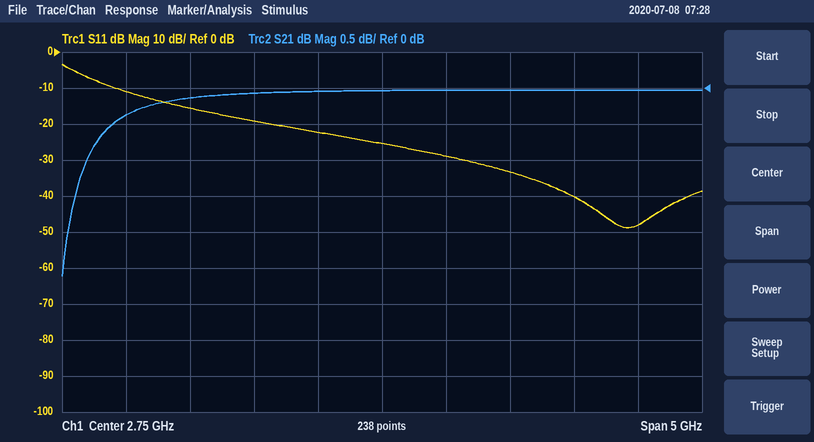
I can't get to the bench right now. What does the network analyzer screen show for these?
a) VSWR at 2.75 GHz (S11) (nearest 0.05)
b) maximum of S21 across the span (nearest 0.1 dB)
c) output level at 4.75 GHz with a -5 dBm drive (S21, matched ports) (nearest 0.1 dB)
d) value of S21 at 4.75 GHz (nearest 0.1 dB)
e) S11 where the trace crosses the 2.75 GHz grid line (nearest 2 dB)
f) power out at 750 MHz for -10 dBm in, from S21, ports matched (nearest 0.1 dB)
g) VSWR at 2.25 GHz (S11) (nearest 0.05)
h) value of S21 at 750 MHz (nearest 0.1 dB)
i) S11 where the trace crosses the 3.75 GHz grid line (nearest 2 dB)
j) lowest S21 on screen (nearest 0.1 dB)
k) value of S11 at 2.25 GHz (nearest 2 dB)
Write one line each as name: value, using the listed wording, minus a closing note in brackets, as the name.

VSWR at 2.75 GHz (S11): 1.10
maximum of S21 across the span: 0.0 dB
output level at 4.75 GHz with a -5 dBm drive (S21, matched ports): -5.0 dBm
value of S21 at 4.75 GHz: 0.0 dB
S11 where the trace crosses the 2.75 GHz grid line: -26 dB
power out at 750 MHz for -10 dBm in, from S21, ports matched: -10.4 dBm
VSWR at 2.25 GHz (S11): 1.15
value of S21 at 750 MHz: -0.4 dB
S11 where the trace crosses the 3.75 GHz grid line: -34 dB
lowest S21 on screen: -2.6 dB
value of S11 at 2.25 GHz: -22 dB
